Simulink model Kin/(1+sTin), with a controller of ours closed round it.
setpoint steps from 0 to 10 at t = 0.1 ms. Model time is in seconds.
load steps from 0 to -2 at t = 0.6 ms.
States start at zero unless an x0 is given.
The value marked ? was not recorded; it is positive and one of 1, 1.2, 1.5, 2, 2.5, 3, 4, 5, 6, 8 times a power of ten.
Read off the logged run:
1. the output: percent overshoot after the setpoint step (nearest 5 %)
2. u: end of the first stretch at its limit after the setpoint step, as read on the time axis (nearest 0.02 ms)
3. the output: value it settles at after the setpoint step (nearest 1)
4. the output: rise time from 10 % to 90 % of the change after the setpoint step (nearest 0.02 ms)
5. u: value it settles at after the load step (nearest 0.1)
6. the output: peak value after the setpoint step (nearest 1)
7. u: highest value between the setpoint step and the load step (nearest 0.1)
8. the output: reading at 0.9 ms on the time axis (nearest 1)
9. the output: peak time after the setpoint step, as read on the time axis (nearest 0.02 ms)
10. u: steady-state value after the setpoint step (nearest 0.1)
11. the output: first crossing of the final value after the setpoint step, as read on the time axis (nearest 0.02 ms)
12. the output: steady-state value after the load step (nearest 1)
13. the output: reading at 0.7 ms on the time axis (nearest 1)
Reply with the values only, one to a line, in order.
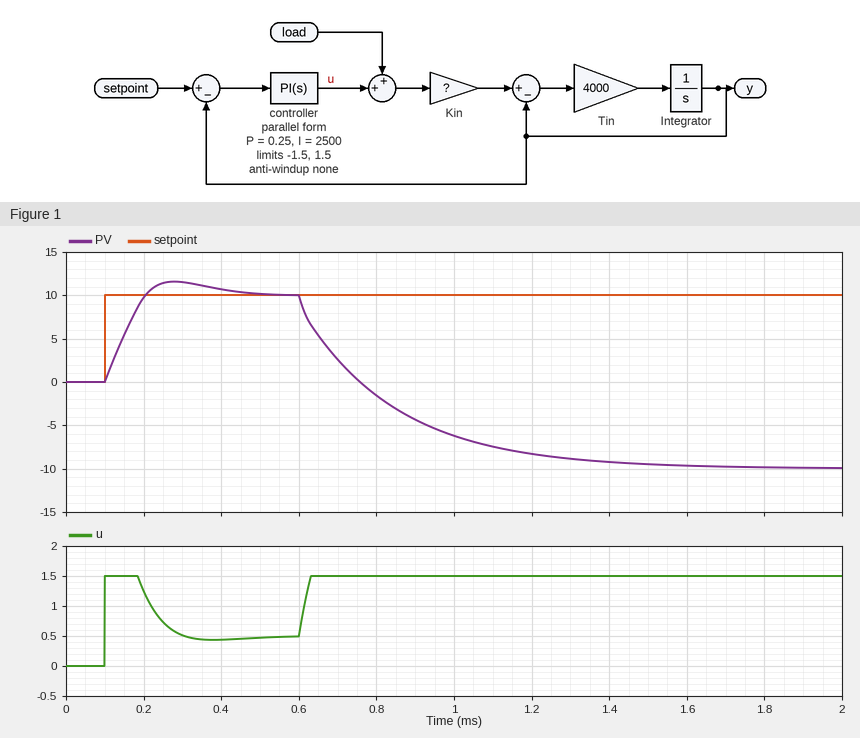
15 %
0.18 ms
10
0.08 ms
1.5
12
1.5
-4
0.28 ms
0.5
0.20 ms
-10
3
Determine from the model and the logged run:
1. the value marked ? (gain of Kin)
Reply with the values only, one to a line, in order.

20
